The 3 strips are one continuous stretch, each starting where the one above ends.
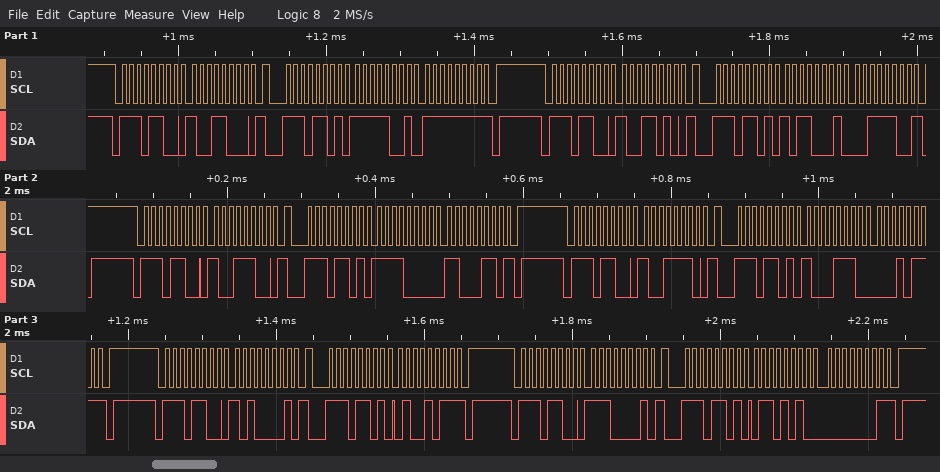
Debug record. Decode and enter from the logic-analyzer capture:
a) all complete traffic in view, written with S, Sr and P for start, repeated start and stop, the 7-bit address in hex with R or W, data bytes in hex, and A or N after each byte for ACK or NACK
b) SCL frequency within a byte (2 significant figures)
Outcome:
S 76W A 98 A Sr 76R A F9 A FF N P S 76W A 9A A Sr 76R A B1 A 3C N P S 76W A 9C A Sr 76R A F0 A C6 N P S 76W A 9E A Sr 76R A 8E A 17 N P S 76W A A1 A Sr 76R A 4B N P S 76W A E1 A Sr 76R A 6A A 01 N P
100 kHz
